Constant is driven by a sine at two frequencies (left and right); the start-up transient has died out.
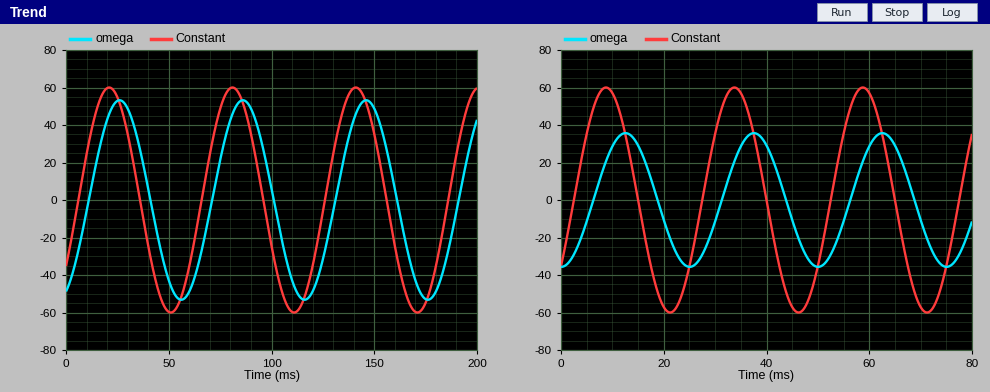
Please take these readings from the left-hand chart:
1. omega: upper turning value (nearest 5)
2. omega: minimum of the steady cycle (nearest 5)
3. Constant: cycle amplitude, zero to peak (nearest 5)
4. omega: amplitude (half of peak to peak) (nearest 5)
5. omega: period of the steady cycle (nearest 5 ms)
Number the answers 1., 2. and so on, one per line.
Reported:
1. 55
2. -55
3. 60
4. 55
5. 60 ms
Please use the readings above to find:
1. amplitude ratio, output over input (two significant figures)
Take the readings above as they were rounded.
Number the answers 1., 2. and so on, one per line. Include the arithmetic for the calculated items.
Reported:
1. 55 / 60 = 0.92
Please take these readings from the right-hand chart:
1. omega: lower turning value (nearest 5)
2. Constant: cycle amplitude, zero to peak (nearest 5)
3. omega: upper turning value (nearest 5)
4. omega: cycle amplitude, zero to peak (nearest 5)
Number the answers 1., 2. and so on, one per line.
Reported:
1. -35
2. 60
3. 35
4. 35
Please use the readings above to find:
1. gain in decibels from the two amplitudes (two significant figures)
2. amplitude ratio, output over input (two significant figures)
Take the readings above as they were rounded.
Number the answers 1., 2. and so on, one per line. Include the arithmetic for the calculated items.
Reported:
1. 20 log10(35 / 60) = -4.7 dB
2. 35 / 60 = 0.58
